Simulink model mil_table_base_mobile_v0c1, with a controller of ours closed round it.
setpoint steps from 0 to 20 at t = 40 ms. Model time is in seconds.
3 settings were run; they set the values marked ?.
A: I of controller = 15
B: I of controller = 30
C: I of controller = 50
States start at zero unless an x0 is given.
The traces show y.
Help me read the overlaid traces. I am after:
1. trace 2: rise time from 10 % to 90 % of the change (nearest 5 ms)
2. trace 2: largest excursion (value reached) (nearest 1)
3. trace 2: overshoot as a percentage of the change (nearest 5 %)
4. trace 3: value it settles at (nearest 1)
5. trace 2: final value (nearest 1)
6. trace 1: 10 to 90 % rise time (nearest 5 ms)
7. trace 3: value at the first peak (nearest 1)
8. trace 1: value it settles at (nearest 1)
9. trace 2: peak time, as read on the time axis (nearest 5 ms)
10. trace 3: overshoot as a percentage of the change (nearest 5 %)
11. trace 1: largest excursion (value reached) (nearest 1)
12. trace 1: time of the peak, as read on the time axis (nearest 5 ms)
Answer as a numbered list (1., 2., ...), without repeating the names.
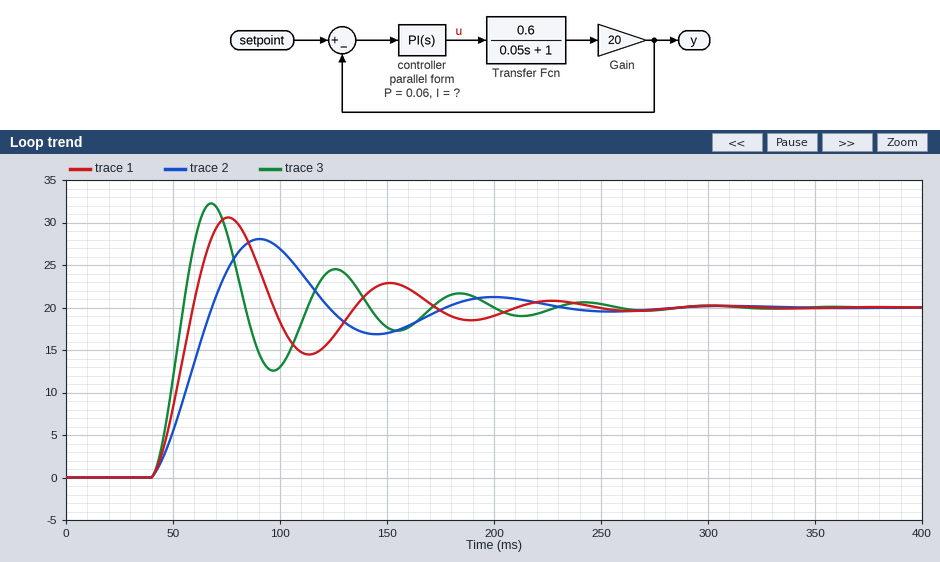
1. 20 ms
2. 28
3. 40 %
4. 20
5. 20
6. 15 ms
7. 32
8. 20
9. 90 ms
10. 60 %
11. 31
12. 75 ms
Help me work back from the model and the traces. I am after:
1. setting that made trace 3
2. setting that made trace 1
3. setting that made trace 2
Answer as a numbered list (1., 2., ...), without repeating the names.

1. C
2. B
3. A
